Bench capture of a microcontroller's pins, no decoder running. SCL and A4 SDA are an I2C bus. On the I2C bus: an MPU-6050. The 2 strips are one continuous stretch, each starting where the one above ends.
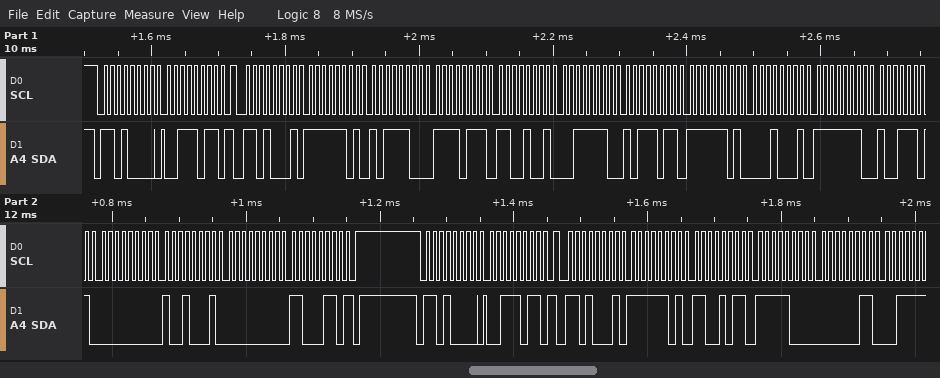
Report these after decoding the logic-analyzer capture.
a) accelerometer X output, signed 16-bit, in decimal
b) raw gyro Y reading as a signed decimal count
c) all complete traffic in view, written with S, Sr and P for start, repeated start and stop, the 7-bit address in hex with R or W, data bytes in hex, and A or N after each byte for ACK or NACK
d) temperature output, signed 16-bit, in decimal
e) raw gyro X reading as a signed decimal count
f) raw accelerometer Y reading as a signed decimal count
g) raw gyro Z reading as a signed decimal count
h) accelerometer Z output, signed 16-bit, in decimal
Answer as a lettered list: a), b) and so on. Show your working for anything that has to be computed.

a) 0xFDBC = -580
b) 0x0091 = 145
c) S 68W A 3B A Sr 68R A FD A BC A F7 A C9 A 3E A BB A FD A 11 A FE A 9D A 00 A 91 A 00 A C6 N P S 68W A 3B A Sr 68R A FD A CB A F8 A 03 A
d) 0xFD11 = -751
e) 0xFE9D = -355
f) 0xF7C9 = -2103
g) 0x00C6 = 198
h) 0x3EBB = 16059
